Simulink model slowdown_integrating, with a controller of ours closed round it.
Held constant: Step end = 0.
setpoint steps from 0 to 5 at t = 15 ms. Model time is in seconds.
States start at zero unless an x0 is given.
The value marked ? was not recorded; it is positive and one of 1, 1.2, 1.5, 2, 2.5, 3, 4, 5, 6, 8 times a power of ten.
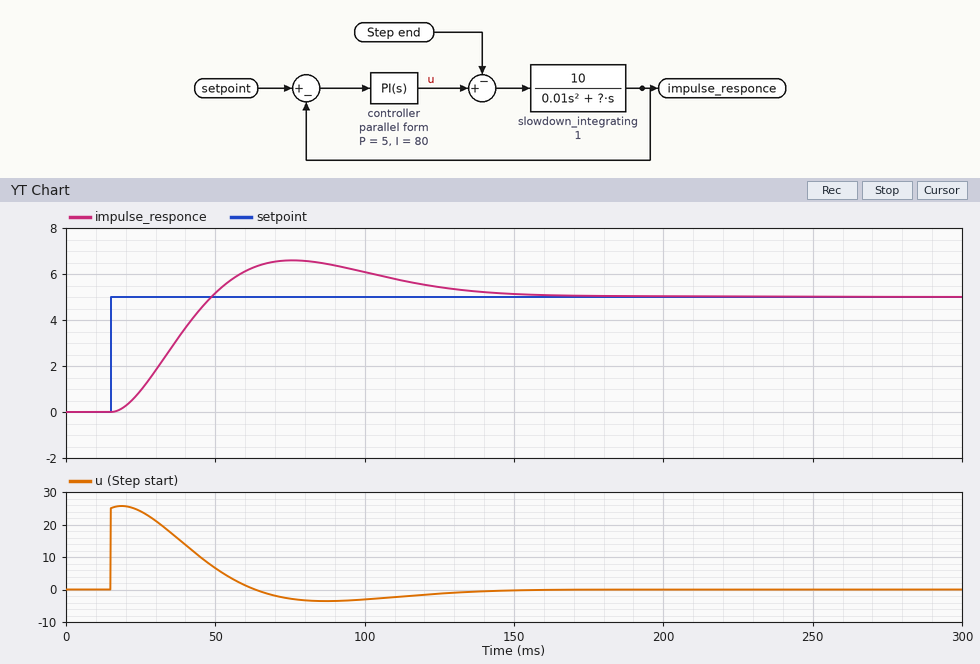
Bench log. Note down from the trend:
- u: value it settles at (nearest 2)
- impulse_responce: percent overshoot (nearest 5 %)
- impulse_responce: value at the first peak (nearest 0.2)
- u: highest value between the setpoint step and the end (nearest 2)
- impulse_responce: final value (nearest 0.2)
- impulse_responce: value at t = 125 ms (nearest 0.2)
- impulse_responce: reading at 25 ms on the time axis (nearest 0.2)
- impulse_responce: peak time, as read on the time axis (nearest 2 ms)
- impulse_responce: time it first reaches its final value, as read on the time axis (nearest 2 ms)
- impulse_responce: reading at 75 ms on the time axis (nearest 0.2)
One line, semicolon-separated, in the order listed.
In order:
0; 30 %; 6.6; 26; 5.0; 5.4; 1.0; 76 ms; 48 ms; 6.6
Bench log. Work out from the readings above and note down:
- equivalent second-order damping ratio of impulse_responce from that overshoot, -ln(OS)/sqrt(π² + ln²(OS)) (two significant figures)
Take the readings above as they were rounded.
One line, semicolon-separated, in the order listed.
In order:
0.36
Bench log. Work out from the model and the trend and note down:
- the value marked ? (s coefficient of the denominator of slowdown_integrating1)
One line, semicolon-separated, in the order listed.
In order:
1
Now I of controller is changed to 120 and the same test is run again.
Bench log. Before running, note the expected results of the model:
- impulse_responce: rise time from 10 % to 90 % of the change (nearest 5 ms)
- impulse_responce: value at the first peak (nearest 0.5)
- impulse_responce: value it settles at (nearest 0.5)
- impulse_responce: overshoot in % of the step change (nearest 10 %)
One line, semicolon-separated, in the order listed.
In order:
20 ms; 7.0; 5.0; 40 %
